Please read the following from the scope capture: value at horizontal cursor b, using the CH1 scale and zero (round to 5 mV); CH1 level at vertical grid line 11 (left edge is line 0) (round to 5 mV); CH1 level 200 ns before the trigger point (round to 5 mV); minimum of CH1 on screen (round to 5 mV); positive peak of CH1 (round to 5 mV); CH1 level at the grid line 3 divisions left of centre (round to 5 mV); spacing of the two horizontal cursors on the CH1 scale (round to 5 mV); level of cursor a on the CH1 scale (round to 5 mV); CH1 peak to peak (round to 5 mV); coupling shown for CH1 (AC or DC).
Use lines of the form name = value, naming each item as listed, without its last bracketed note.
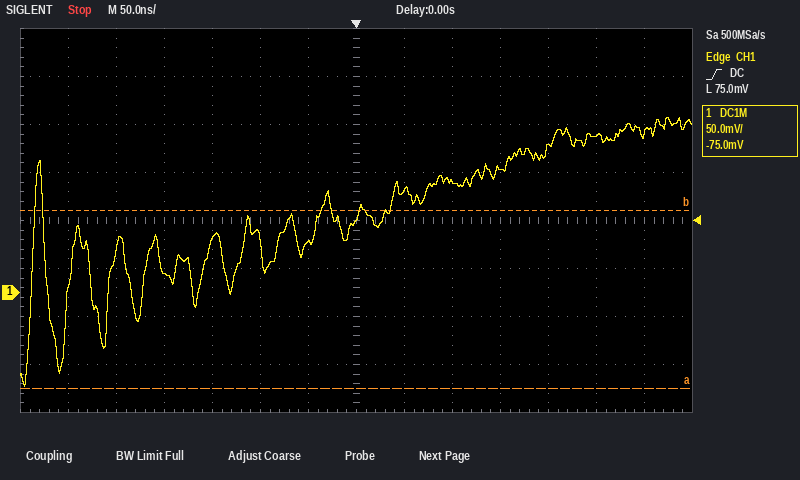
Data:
value at horizontal cursor b, using the CH1 scale and zero = 85 mV
CH1 level at vertical grid line 11 (left edge is line 0) = 150 mV
CH1 level 200 ns before the trigger point = 20 mV
minimum of CH1 on screen = -100 mV
positive peak of CH1 = 180 mV
CH1 level at the grid line 3 divisions left of centre = 55 mV
spacing of the two horizontal cursors on the CH1 scale = 185 mV
level of cursor a on the CH1 scale = -100 mV
CH1 peak to peak = 280 mV
coupling shown for CH1 = DC
